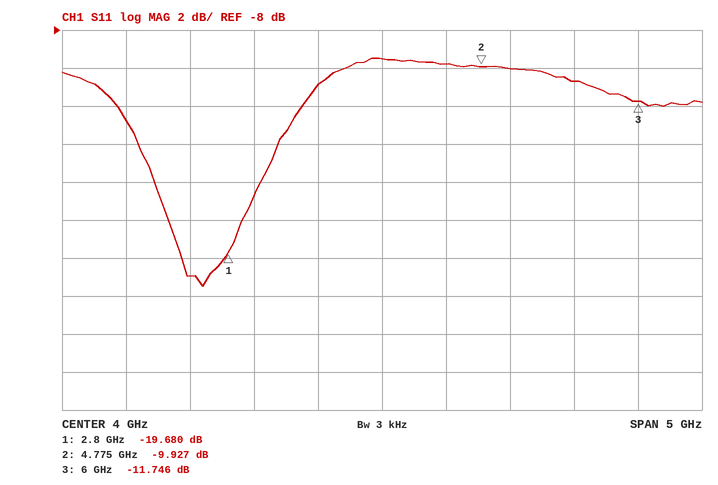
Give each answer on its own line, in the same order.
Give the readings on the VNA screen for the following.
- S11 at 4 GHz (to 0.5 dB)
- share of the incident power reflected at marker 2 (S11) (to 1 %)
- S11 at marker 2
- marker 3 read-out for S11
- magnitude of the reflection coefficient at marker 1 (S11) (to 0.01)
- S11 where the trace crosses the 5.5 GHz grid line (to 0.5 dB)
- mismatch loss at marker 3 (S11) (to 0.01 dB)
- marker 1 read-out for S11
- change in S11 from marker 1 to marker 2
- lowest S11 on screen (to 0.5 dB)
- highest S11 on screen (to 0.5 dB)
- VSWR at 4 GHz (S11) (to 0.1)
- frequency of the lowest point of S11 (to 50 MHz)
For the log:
-9.5 dB
10 %
-9.927 dB
-11.746 dB
0.10
-10.5 dB
0.30 dB
-19.680 dB
9.753 dB
-21.5 dB
-9.5 dB
2.0
2.60 GHz
